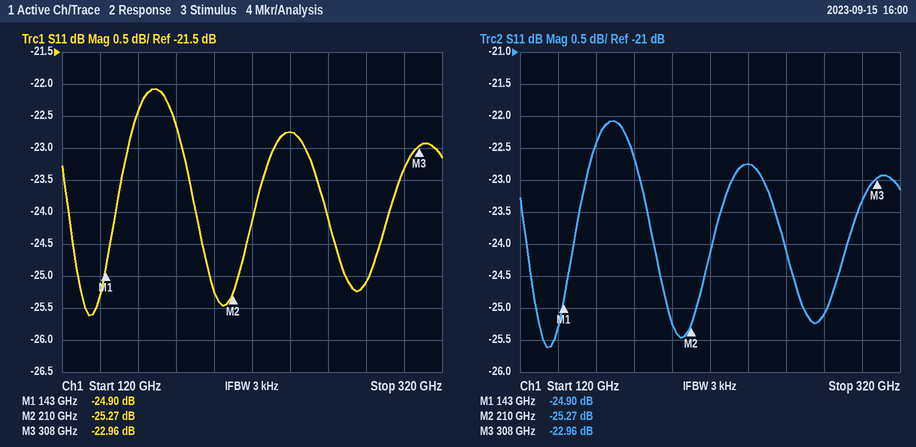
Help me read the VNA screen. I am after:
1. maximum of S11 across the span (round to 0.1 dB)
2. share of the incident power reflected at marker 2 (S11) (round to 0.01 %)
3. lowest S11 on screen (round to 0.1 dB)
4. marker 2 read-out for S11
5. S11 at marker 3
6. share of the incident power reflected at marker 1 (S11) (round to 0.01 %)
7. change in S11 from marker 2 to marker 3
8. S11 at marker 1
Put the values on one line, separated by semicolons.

-22.1 dB; 0.30 %; -25.6 dB; -25.27 dB; -22.96 dB; 0.32 %; 2.31 dB; -24.90 dB
